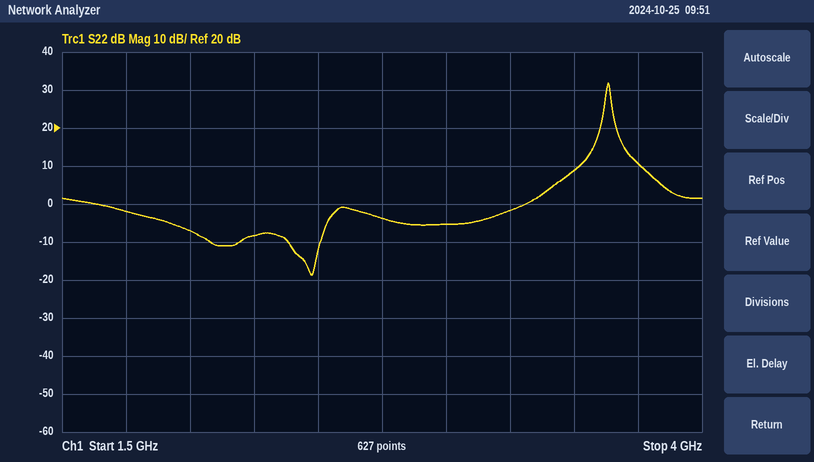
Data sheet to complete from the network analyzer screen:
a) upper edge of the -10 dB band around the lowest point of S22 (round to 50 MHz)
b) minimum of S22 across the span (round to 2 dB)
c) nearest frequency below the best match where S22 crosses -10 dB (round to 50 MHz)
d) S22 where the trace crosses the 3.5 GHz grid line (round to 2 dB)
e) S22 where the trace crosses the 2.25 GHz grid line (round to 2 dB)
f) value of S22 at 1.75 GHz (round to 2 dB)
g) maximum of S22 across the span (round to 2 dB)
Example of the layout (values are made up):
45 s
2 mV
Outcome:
2.50 GHz
-18 dB
2.40 GHz
8 dB
-8 dB
-2 dB
32 dB
